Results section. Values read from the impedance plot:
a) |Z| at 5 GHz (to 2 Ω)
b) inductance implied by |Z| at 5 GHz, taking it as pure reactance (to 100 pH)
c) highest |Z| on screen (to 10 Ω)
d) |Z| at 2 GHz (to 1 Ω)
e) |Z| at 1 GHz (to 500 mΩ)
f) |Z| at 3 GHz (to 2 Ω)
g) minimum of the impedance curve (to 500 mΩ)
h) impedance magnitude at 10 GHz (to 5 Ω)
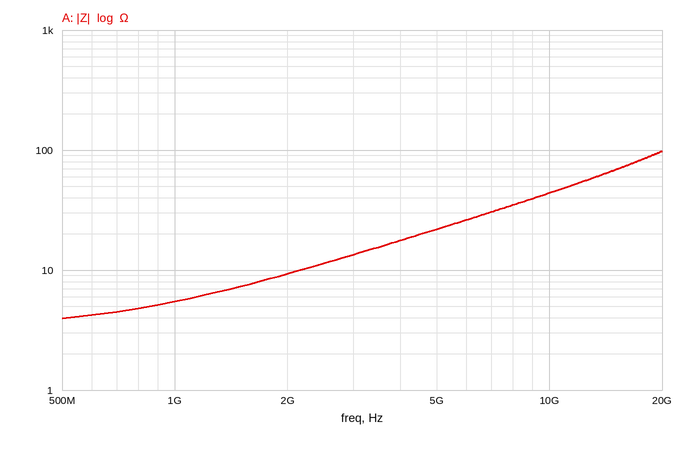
22 Ω
700 pH
100 Ω
9 Ω
5.5 Ω
14 Ω
4.0 Ω
45 Ω
